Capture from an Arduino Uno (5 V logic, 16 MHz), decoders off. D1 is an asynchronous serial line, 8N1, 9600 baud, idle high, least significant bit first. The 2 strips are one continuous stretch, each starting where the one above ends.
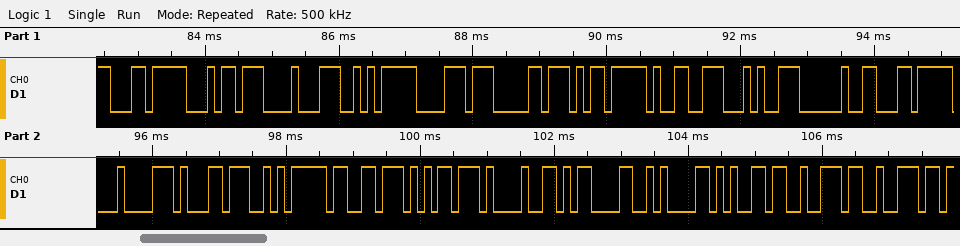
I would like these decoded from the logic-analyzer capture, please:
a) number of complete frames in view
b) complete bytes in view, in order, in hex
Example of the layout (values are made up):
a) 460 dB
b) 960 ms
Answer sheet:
a) 22
b) EC B4 88 EA B8 B0 ED 99 94 20 EC 84 B1 EA B3 B5 21 0D 0A 65 72 72
